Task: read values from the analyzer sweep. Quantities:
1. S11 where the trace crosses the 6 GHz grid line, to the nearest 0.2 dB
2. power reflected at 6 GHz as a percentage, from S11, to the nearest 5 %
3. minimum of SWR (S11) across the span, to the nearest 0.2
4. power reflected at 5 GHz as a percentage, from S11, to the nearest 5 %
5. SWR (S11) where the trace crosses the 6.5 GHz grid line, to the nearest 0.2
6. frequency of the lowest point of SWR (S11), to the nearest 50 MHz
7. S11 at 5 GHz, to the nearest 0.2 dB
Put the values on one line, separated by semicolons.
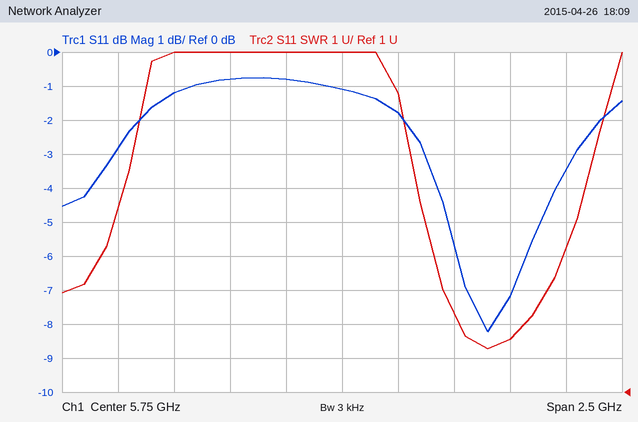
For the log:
-1.8 dB; 65 %; 2.2; 75 %; 2.6; 6.40 GHz; -1.2 dB
